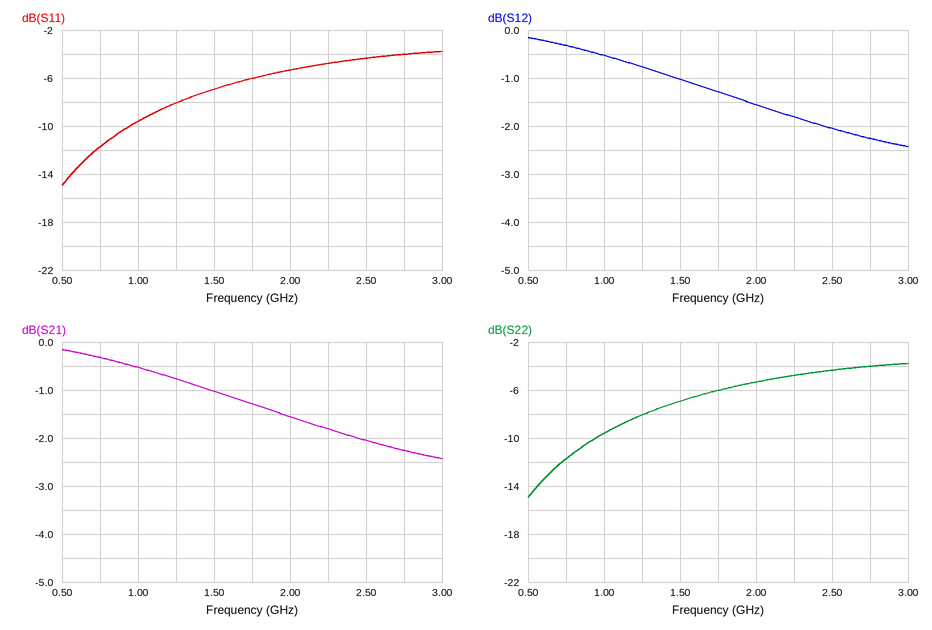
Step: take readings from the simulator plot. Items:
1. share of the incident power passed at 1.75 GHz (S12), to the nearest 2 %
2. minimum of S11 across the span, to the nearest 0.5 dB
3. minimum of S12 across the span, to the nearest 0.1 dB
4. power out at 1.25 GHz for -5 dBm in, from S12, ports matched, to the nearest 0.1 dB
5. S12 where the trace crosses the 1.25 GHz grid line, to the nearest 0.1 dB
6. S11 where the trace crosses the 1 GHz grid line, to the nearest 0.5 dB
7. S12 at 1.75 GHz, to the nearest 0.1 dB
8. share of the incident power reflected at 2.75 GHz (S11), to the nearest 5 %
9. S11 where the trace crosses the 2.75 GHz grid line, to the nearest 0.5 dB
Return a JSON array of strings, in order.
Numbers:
["74 %", "-15.0 dB", "-2.4 dB", "-5.8 dBm", "-0.8 dB", "-9.5 dB", "-1.3 dB", "40 %", "-4.0 dB"]
